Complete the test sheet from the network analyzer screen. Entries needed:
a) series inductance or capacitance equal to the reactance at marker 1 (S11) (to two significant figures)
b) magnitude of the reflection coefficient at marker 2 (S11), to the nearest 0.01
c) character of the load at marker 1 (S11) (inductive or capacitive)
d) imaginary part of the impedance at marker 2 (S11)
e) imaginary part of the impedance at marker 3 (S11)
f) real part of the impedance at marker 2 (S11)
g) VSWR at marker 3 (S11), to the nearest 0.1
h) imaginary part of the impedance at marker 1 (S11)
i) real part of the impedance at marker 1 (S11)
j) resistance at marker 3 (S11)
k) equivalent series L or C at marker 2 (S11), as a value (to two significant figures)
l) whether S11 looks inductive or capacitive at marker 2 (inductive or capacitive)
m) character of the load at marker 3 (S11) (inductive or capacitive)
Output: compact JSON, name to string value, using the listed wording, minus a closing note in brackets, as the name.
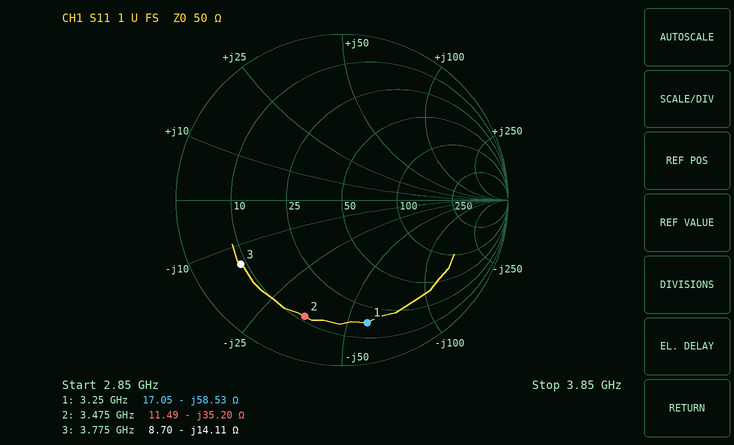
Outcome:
{"series inductance or capacitance equal to the reactance at marker 1 (S11)": "840 fF", "magnitude of the reflection coefficient at marker 2 (S11), to the nearest 0.01": "0.74", "character of the load at marker 1 (S11)": "capacitive", "imaginary part of the impedance at marker 2": "-35.20 Ω", "imaginary part of the impedance at marker 3": "-14.11 Ω", "real part of the impedance at marker 2": "11.49 Ω", "VSWR at marker 3 (S11), to the nearest 0.1": "6.2", "imaginary part of the impedance at marker 1": "-58.53 Ω", "real part of the impedance at marker 1": "17.05 Ω", "resistance at marker 3": "8.70 Ω", "equivalent series L or C at marker 2 (S11), as a value": "1.3 pF", "whether S11 looks inductive or capacitive at marker 2": "capacitive", "character of the load at marker 3 (S11)": "capacitive"}
